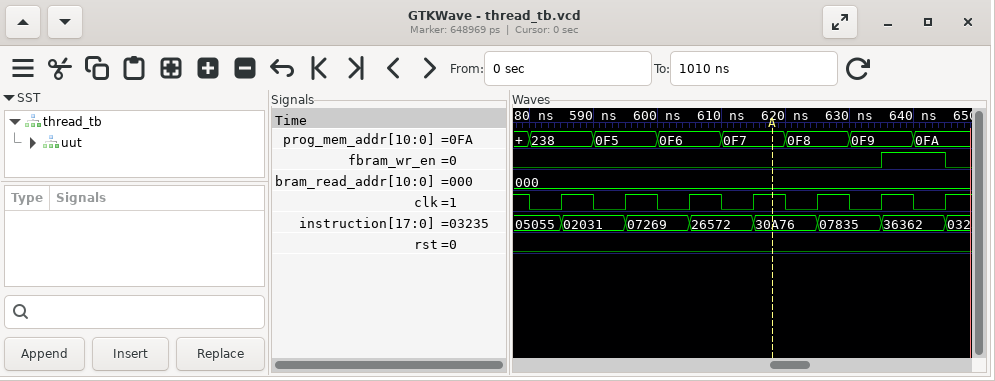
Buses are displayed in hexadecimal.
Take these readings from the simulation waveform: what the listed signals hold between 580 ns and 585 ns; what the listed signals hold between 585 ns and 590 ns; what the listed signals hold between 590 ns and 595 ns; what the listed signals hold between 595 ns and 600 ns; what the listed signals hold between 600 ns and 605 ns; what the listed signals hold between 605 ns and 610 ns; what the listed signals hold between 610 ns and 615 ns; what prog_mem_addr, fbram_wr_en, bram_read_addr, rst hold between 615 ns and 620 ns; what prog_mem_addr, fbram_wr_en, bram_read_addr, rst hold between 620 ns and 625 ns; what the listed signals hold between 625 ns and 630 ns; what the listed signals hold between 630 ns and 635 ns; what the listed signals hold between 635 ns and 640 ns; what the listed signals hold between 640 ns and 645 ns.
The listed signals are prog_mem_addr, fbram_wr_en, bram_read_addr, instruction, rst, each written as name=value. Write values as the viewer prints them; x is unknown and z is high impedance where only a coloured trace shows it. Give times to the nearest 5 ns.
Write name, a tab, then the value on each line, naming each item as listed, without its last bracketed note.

what the listed signals hold between 580 ns and 585 ns	prog_mem_addr=238, fbram_wr_en=0, bram_read_addr=000, instruction=05055, rst=0
what the listed signals hold between 585 ns and 590 ns	prog_mem_addr=238, fbram_wr_en=0, bram_read_addr=000, instruction=02031, rst=0
what the listed signals hold between 590 ns and 595 ns	prog_mem_addr=0F5, fbram_wr_en=0, bram_read_addr=000, instruction=02031, rst=0
what the listed signals hold between 595 ns and 600 ns	prog_mem_addr=0F5, fbram_wr_en=0, bram_read_addr=000, instruction=07269, rst=0
what the listed signals hold between 600 ns and 605 ns	prog_mem_addr=0F6, fbram_wr_en=0, bram_read_addr=000, instruction=07269, rst=0
what the listed signals hold between 605 ns and 610 ns	prog_mem_addr=0F6, fbram_wr_en=0, bram_read_addr=000, instruction=26572, rst=0
what the listed signals hold between 610 ns and 615 ns	prog_mem_addr=0F7, fbram_wr_en=0, bram_read_addr=000, instruction=26572, rst=0
what prog_mem_addr, fbram_wr_en, bram_read_addr, rst hold between 615 ns and 620 ns	prog_mem_addr=0F7, fbram_wr_en=0, bram_read_addr=000, rst=0
what prog_mem_addr, fbram_wr_en, bram_read_addr, rst hold between 620 ns and 625 ns	prog_mem_addr=0F8, fbram_wr_en=0, bram_read_addr=000, rst=0
what the listed signals hold between 625 ns and 630 ns	prog_mem_addr=0F8, fbram_wr_en=0, bram_read_addr=000, instruction=07835, rst=0
what the listed signals hold between 630 ns and 635 ns	prog_mem_addr=0F9, fbram_wr_en=0, bram_read_addr=000, instruction=07835, rst=0
what the listed signals hold between 635 ns and 640 ns	prog_mem_addr=0F9, fbram_wr_en=1, bram_read_addr=000, instruction=36362, rst=0
what the listed signals hold between 640 ns and 645 ns	prog_mem_addr=0FA, fbram_wr_en=1, bram_read_addr=000, instruction=36362, rst=0
